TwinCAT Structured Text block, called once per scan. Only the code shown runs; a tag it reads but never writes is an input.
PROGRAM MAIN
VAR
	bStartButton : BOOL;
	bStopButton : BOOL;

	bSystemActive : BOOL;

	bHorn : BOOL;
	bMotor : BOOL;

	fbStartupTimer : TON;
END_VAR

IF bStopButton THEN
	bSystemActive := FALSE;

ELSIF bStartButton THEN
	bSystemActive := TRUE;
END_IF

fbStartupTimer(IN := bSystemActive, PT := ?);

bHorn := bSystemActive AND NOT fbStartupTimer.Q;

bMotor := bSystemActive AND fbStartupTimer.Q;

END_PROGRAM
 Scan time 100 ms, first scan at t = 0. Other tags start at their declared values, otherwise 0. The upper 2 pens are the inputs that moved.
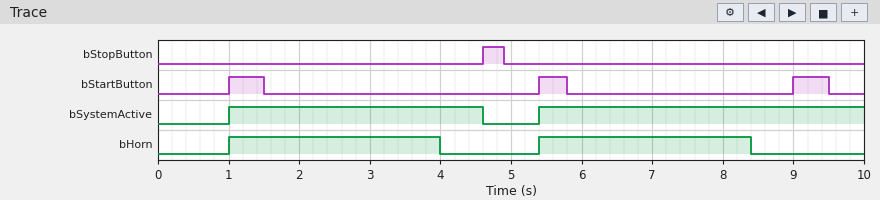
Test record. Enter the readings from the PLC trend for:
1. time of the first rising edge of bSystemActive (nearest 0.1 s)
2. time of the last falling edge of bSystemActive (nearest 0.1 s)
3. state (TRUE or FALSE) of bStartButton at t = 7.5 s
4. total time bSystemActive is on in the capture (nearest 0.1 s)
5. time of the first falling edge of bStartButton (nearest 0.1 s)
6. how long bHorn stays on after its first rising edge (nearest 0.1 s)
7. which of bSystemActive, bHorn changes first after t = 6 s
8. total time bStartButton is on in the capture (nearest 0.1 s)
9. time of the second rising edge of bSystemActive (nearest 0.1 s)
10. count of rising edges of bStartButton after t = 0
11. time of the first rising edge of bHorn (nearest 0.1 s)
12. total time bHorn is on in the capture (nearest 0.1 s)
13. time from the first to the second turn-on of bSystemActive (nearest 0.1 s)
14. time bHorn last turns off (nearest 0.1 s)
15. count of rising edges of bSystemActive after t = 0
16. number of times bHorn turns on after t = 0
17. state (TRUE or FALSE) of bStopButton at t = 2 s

1.0 s
4.6 s
FALSE
8.2 s
1.5 s
3.0 s
bHorn
1.4 s
5.4 s
3
1.0 s
6.0 s
4.4 s
8.4 s
2
2
FALSE
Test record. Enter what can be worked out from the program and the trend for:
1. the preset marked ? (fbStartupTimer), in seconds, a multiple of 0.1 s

3.0 s
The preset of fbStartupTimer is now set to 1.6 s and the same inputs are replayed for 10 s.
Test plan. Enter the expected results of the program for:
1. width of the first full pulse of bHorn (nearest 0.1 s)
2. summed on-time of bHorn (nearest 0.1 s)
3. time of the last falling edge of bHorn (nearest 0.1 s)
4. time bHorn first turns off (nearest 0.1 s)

1.6 s
3.2 s
7.0 s
2.6 s
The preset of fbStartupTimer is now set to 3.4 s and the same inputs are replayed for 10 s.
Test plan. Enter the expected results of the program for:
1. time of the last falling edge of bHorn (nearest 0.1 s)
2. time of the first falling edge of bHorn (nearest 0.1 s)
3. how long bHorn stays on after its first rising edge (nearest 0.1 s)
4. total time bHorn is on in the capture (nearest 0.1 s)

8.8 s
4.4 s
3.4 s
6.8 s
